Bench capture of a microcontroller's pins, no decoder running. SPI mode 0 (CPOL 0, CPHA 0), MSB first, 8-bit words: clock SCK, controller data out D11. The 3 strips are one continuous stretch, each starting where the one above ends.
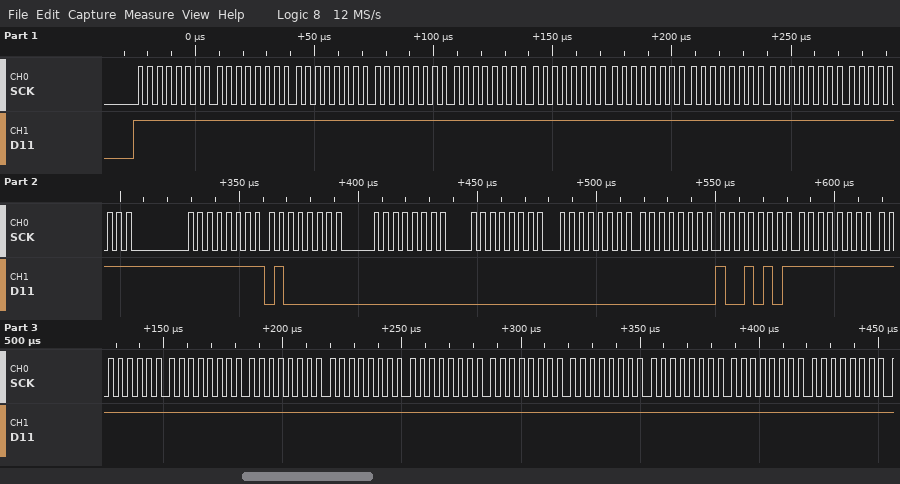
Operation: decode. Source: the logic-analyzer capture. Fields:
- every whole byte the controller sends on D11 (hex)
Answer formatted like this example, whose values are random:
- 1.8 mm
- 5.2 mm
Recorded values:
- 0xFF 0xFF 0xFF 0xFF 0xFF 0xFF 0xFF 0xFF 0xFF 0xFF 0xFF 0x40 0x00 0x00 0x00 0x00 0x95 0xFF 0xFF 0xFF 0xFF 0xFF 0xFF 0xFF 0xFF 0xFF 0xFF 0xFF
